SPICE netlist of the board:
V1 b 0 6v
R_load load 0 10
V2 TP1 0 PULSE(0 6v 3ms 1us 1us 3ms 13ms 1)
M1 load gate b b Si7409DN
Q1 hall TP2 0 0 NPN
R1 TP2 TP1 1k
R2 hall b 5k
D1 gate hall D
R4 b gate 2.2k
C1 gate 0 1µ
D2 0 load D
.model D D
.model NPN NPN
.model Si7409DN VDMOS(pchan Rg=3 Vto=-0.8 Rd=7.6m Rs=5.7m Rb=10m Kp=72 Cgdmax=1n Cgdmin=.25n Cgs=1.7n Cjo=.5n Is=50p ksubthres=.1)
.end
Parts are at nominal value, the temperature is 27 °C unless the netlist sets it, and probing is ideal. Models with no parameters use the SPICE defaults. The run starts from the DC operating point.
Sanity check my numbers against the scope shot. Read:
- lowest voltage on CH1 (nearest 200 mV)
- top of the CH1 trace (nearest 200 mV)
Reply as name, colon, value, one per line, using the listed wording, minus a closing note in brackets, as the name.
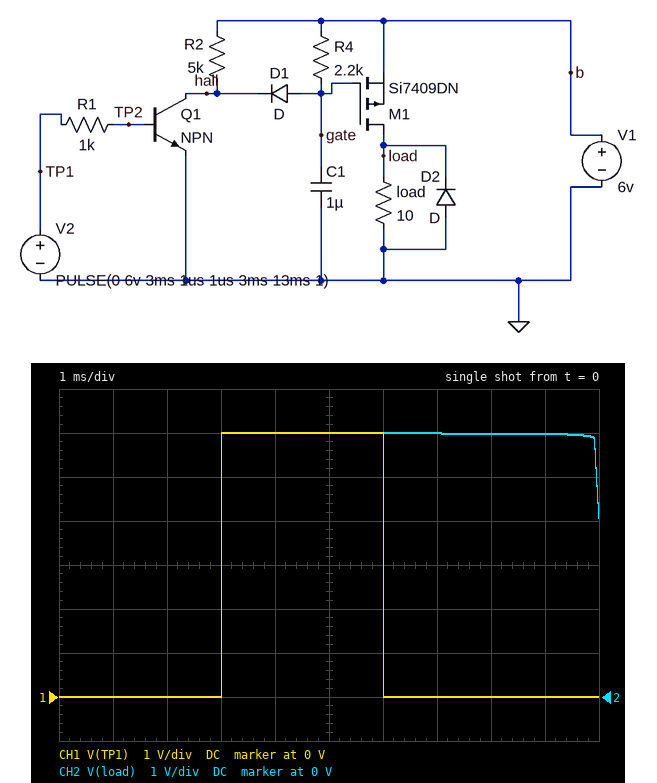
lowest voltage on CH1: 0 V
top of the CH1 trace: 6.0 V
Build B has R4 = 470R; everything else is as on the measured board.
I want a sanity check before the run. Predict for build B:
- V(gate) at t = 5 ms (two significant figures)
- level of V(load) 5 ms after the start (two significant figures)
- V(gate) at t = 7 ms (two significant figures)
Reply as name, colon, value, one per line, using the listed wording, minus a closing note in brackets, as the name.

V(gate) at t = 5 ms: 760 mV
level of V(load) 5 ms after the start: 6.0 V
V(gate) at t = 7 ms: 5.4 V
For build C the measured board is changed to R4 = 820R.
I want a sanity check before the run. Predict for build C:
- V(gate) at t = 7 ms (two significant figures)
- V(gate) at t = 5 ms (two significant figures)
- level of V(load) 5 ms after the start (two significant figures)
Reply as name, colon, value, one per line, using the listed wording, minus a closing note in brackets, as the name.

V(gate) at t = 7 ms: 4.4 V
V(gate) at t = 5 ms: 740 mV
level of V(load) 5 ms after the start: 6.0 V
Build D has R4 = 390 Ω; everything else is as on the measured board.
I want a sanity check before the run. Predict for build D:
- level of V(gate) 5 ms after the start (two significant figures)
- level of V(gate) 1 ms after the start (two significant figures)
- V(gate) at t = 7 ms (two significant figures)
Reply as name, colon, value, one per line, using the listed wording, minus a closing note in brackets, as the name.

level of V(gate) 5 ms after the start: 760 mV
level of V(gate) 1 ms after the start: 6.0 V
V(gate) at t = 7 ms: 5.6 V
